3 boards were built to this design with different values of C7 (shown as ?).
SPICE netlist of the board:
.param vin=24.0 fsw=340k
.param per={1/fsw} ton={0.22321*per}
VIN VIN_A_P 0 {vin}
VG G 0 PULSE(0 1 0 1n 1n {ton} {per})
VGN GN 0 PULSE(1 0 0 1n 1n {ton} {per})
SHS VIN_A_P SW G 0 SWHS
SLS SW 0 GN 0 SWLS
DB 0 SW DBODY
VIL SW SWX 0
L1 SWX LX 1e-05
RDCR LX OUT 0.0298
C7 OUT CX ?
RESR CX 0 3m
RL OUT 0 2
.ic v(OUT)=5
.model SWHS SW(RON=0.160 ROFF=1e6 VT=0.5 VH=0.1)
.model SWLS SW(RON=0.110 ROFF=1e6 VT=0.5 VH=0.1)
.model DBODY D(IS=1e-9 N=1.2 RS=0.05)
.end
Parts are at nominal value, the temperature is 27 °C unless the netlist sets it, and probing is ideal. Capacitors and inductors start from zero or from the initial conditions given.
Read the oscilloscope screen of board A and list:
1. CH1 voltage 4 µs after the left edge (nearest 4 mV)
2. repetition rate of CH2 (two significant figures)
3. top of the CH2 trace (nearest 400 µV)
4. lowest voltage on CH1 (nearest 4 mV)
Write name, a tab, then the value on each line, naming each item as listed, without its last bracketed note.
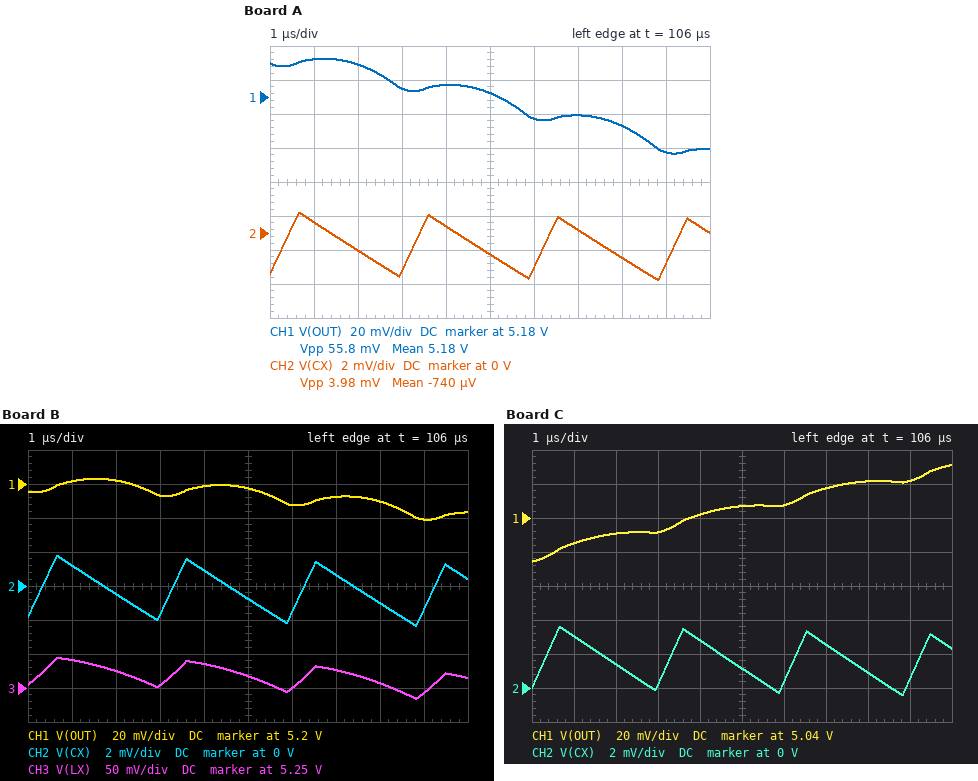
CH1 voltage 4 µs after the left edge	5.188 V
repetition rate of CH2	340 kHz
top of the CH2 trace	1.2 mV
lowest voltage on CH1	5.148 V
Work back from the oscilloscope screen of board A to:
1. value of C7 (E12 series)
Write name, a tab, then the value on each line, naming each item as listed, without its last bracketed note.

value of C7	47 µF
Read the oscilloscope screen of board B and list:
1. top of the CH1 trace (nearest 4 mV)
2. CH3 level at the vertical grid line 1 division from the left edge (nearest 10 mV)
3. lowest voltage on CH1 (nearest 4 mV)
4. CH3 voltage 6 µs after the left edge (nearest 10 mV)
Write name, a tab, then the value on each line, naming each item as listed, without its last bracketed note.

top of the CH1 trace	5.204 V
CH3 level at the vertical grid line 1 division from the left edge	5.29 V
lowest voltage on CH1	5.180 V
CH3 voltage 6 µs after the left edge	5.25 V
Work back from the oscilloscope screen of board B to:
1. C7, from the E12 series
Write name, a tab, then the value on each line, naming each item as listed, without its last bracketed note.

C7, from the E12 series	56 µF
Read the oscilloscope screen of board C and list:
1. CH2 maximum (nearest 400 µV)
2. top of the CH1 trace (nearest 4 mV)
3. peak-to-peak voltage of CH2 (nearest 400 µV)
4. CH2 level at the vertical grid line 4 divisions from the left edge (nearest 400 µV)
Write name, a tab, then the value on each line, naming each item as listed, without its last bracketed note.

CH2 maximum	3.6 mV
top of the CH1 trace	5.072 V
peak-to-peak voltage of CH2	4.0 mV
CH2 level at the vertical grid line 4 divisions from the left edge	2.8 mV
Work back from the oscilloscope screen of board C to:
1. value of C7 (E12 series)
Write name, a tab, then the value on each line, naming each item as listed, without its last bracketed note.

value of C7	100 µF
